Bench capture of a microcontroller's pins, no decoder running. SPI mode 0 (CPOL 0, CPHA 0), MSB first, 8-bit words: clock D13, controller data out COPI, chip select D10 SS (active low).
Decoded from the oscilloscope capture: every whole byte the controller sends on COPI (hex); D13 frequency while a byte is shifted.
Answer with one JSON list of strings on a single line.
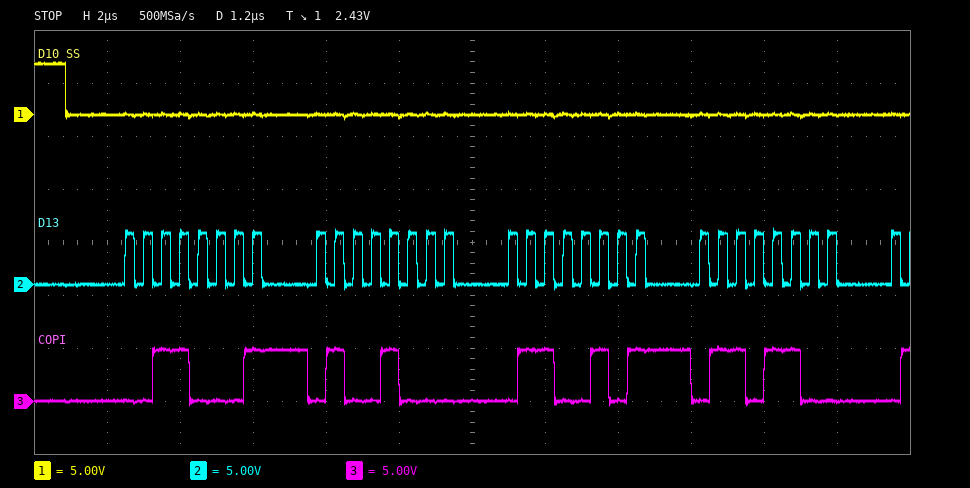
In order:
["31 48 65 6C", "2 MHz"]
